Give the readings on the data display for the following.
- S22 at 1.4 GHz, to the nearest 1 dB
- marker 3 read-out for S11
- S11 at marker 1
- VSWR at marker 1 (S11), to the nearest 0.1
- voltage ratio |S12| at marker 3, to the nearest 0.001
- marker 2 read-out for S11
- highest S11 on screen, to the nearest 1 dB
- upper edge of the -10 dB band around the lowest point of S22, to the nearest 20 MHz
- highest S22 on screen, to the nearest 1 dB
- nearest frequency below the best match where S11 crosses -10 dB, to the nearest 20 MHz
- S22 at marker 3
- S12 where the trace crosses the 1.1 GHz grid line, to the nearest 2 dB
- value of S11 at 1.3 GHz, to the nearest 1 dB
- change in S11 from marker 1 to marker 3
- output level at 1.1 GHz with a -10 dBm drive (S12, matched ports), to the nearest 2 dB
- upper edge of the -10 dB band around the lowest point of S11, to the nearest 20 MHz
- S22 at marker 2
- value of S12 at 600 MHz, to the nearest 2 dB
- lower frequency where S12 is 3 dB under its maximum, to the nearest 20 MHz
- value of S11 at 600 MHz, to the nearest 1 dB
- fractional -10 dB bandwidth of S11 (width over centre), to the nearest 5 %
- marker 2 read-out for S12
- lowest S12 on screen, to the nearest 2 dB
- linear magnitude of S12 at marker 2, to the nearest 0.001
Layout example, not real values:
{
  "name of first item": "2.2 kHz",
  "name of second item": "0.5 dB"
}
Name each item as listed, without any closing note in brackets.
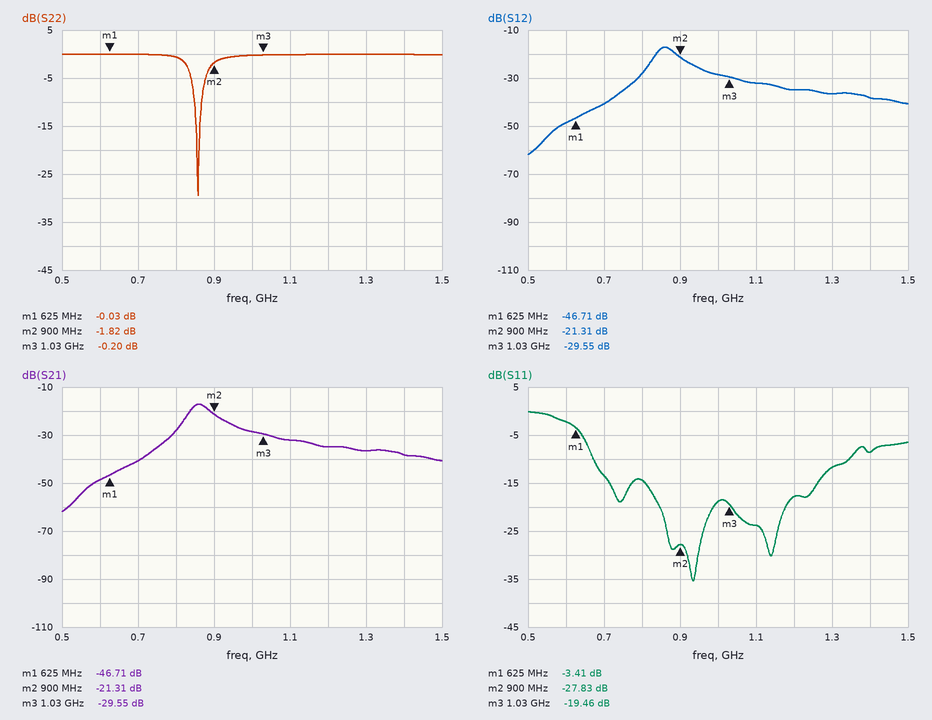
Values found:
{
  "S22 at 1.4 GHz, to the nearest 1 dB": "0 dB",
  "marker 3 read-out for S11": "-19.46 dB",
  "S11 at marker 1": "-3.41 dB",
  "VSWR at marker 1 (S11), to the nearest 0.1": "5.2",
  "voltage ratio |S12| at marker 3, to the nearest 0.001": "0.033",
  "marker 2 read-out for S11": "-27.83 dB",
  "highest S11 on screen, to the nearest 1 dB": "0 dB",
  "upper edge of the -10 dB band around the lowest point of S22, to the nearest 20 MHz": "860 MHz",
  "highest S22 on screen, to the nearest 1 dB": "0 dB",
  "nearest frequency below the best match where S11 crosses -10 dB, to the nearest 20 MHz": "680 MHz",
  "S22 at marker 3": "-0.20 dB",
  "S12 where the trace crosses the 1.1 GHz grid line, to the nearest 2 dB": "-32 dB",
  "value of S11 at 1.3 GHz, to the nearest 1 dB": "-12 dB",
  "change in S11 from marker 1 to marker 3": "-16.05 dB",
  "output level at 1.1 GHz with a -10 dBm drive (S12, matched ports), to the nearest 2 dB": "-42 dBm",
  "upper edge of the -10 dB band around the lowest point of S11, to the nearest 20 MHz": "1.34 GHz",
  "S22 at marker 2": "-1.82 dB",
  "value of S12 at 600 MHz, to the nearest 2 dB": "-48 dB",
  "lower frequency where S12 is 3 dB under its maximum, to the nearest 20 MHz": "840 MHz",
  "value of S11 at 600 MHz, to the nearest 1 dB": "-2 dB",
  "fractional -10 dB bandwidth of S11 (width over centre), to the nearest 5 %": "65 %",
  "marker 2 read-out for S12": "-21.31 dB",
  "lowest S12 on screen, to the nearest 2 dB": "-62 dB",
  "linear magnitude of S12 at marker 2, to the nearest 0.001": "0.086"
}
